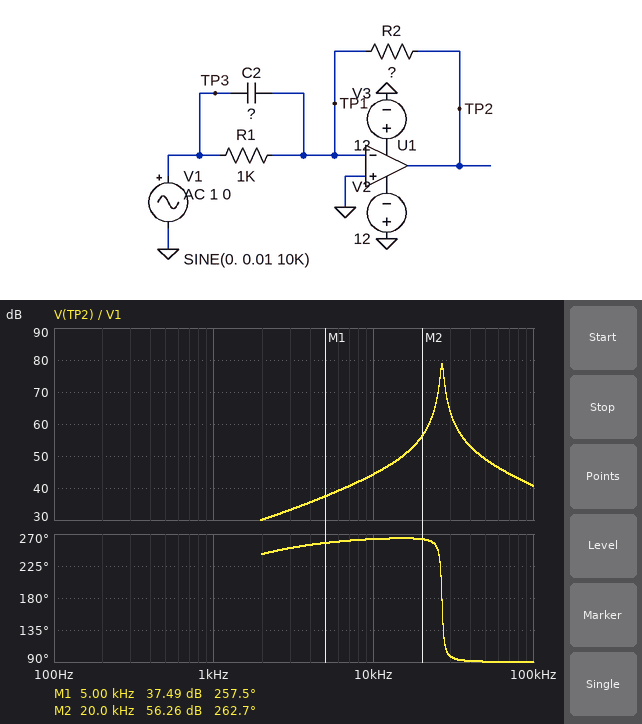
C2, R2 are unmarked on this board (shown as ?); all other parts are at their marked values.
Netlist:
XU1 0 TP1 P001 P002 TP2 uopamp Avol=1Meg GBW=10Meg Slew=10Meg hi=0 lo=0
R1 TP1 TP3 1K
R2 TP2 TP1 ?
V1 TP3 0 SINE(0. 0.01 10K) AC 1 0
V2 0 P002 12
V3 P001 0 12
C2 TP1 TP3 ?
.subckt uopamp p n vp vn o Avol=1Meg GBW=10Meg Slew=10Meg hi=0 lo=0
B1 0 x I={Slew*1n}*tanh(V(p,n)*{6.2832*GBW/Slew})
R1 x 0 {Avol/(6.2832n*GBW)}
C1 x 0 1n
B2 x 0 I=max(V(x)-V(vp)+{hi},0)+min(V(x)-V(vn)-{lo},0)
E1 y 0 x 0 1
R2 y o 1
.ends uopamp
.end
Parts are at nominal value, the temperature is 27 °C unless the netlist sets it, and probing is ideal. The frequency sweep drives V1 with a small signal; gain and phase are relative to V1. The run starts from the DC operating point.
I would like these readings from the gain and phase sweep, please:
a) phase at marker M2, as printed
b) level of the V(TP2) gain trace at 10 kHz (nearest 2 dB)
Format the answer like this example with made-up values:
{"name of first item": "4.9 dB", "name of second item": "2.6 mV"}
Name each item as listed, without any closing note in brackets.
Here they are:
{"phase at marker M2, as printed": "262.7 deg", "level of the V(TP2) gain trace at 10 kHz": "44 dB"}
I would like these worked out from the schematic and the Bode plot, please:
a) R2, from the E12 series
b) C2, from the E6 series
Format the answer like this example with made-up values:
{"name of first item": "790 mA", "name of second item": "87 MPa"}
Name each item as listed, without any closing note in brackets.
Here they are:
{"R2, from the E12 series": "15 kΩ", "C2, from the E6 series": "150 nF"}
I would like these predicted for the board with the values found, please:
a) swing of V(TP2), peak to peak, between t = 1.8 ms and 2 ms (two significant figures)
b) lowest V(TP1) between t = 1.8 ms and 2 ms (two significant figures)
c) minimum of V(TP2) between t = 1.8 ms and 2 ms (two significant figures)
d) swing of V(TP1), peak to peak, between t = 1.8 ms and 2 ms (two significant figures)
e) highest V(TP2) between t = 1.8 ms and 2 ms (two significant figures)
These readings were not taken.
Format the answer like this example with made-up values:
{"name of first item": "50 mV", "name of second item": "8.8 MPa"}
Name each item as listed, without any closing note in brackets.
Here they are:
{"swing of V(TP2), peak to peak, between t = 1.8 ms and 2 ms": "3.3 V", "lowest V(TP1) between t = 1.8 ms and 2 ms": "-1.7 mV", "minimum of V(TP2) between t = 1.8 ms and 2 ms": "-1.7 V", "swing of V(TP1), peak to peak, between t = 1.8 ms and 2 ms": "3.3 mV", "highest V(TP2) between t = 1.8 ms and 2 ms": "1.7 V"}
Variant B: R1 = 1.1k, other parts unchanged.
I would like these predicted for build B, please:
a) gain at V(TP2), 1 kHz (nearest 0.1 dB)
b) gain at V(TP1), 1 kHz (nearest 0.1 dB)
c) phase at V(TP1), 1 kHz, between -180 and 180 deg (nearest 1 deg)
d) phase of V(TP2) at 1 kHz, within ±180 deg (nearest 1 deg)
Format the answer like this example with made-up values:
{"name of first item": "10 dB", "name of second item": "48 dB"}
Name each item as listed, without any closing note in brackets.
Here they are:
{"gain at V(TP2), 1 kHz": "25.9 dB", "gain at V(TP1), 1 kHz": "-54.1 dB", "phase at V(TP1), 1 kHz, between -180 and 180 deg": "135 deg", "phase of V(TP2) at 1 kHz, within ±180 deg": "-134 deg"}
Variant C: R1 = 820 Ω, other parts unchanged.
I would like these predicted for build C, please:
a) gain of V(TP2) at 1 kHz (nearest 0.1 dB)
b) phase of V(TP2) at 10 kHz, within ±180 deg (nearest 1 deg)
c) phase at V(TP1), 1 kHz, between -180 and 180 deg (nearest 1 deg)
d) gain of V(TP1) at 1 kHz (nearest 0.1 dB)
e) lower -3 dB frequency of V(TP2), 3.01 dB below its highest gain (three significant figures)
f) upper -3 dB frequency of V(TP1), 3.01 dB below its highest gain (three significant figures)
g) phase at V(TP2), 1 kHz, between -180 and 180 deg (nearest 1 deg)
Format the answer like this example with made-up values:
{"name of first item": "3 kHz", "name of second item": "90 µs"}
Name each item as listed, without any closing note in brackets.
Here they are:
{"gain of V(TP2) at 1 kHz": "27.3 dB", "phase of V(TP2) at 10 kHz, within ±180 deg": "-99 deg", "phase at V(TP1), 1 kHz, between -180 and 180 deg": "127 deg", "gain of V(TP1) at 1 kHz": "-52.7 dB", "lower -3 dB frequency of V(TP2), 3.01 dB below its highest gain": "25.9 kHz", "upper -3 dB frequency of V(TP1), 3.01 dB below its highest gain": "27.3 kHz", "phase at V(TP2), 1 kHz, between -180 and 180 deg": "-142 deg"}
